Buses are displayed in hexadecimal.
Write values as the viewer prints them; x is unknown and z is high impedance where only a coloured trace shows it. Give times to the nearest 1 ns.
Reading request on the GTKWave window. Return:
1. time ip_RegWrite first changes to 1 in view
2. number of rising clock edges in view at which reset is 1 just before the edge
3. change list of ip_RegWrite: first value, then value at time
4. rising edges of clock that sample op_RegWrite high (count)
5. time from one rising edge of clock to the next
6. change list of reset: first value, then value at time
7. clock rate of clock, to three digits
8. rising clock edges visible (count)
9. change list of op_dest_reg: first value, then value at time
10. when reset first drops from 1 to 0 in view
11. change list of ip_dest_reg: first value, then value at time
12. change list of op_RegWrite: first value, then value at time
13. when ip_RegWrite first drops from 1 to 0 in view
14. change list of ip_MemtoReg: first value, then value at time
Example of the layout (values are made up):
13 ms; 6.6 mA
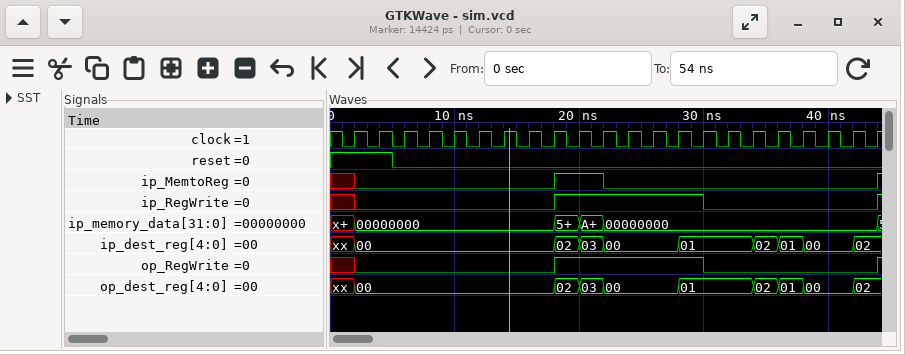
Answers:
18 ns; 2; x, 0 at 2 ns, 1 at 18 ns, 0 at 30 ns, 1 at 44 ns; 6; 2 ns; 1, 0 at 5 ns; 500 MHz; 22; xx, 00 at 2 ns, 02 at 18 ns, 03 at 20 ns, 00 at 22 ns, 01 at 28 ns, 02 at 34 ns, 01 at 36 ns, 00 at 38 ns, 02 at 42 ns; 5 ns; xx, 00 at 2 ns, 02 at 18 ns, 03 at 20 ns, 00 at 22 ns, 01 at 28 ns, 02 at 34 ns, 01 at 36 ns, 00 at 38 ns, 02 at 42 ns; x, 0 at 2 ns, 1 at 18 ns, 0 at 30 ns, 1 at 44 ns; 30 ns; x, 0 at 2 ns, 1 at 18 ns, 0 at 22 ns, 1 at 44 ns
